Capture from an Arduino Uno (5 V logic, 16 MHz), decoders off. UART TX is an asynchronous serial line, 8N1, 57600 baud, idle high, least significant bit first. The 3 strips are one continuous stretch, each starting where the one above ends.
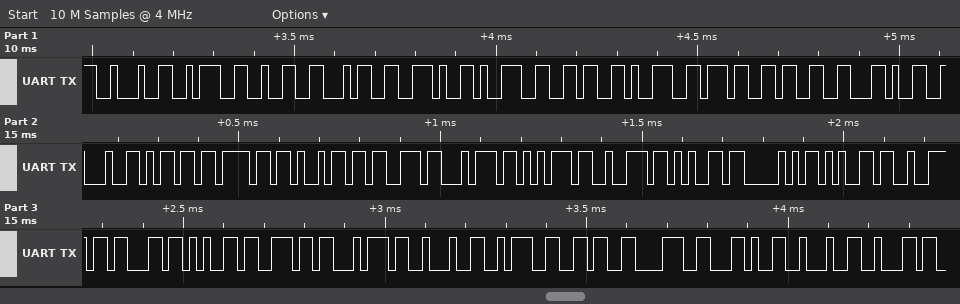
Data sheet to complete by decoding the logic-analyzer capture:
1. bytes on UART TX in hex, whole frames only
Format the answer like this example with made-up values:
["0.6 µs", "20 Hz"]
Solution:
["22 3A 32 34 2E 39 36 39 37 33 2C 22 6D 6F 69 73 74 75 72 65 50 65 72 63 65 6E 74 22 3A 36 38 2C 22 62"]
